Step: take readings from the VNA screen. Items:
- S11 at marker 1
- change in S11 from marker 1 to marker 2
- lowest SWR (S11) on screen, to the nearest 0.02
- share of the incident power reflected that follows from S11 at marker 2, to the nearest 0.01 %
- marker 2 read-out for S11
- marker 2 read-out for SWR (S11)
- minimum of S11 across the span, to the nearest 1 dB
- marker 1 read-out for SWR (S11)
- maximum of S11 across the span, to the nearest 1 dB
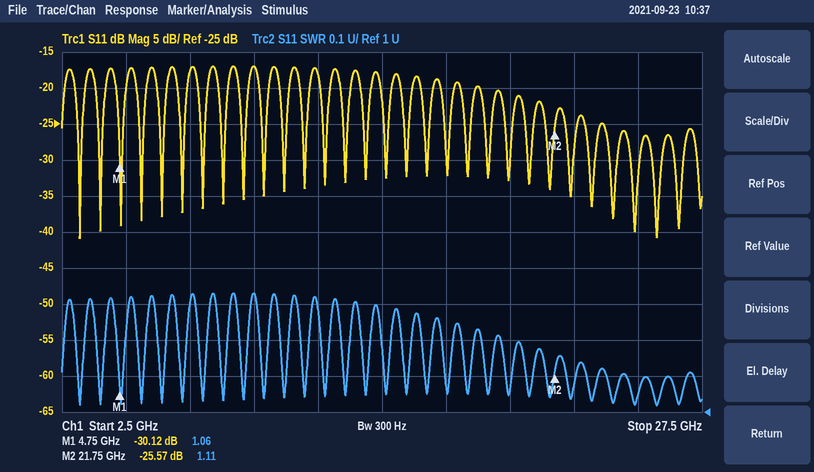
-30.12 dB
4.55 dB
1.02
0.28 %
-25.57 dB
1.11
-41 dB
1.06
-17 dB
